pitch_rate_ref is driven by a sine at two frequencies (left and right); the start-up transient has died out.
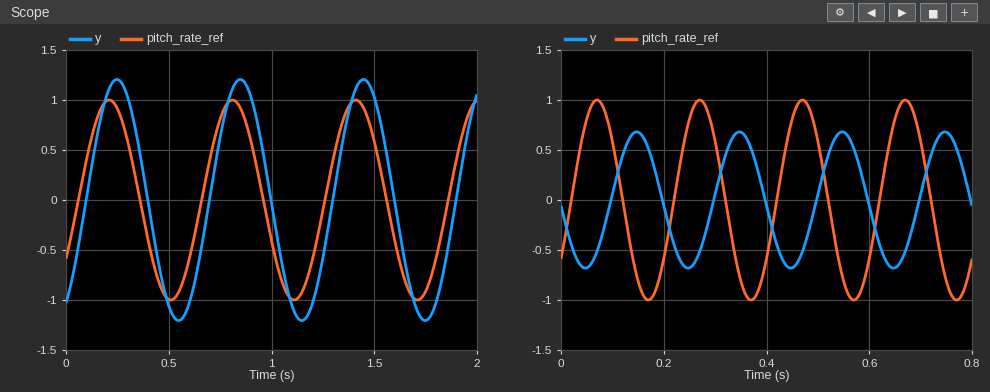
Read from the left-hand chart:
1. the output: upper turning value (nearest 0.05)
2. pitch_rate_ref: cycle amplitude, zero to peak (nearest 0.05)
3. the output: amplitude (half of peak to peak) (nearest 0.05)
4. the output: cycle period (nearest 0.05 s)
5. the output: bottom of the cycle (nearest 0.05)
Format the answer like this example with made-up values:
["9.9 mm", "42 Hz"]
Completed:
["1.20", "1.00", "1.20", "0.60 s", "-1.20"]
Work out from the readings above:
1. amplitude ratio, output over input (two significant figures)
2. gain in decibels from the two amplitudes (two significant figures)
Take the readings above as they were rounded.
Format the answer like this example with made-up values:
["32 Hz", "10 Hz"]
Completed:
["1.2", "1.6 dB"]
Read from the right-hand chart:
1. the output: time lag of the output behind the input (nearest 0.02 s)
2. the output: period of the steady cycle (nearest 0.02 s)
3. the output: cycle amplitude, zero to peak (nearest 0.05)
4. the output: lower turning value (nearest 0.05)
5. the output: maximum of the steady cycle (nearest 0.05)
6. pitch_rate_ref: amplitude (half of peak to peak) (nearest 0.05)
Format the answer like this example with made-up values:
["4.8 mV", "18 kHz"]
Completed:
["0.08 s", "0.20 s", "0.70", "-0.70", "0.70", "1.00"]
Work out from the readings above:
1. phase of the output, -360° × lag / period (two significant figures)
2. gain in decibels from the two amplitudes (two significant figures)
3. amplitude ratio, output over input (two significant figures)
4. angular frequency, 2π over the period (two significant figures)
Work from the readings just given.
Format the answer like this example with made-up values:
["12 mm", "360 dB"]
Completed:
["-140°", "-3.1 dB", "0.70", "31 rad/s"]
